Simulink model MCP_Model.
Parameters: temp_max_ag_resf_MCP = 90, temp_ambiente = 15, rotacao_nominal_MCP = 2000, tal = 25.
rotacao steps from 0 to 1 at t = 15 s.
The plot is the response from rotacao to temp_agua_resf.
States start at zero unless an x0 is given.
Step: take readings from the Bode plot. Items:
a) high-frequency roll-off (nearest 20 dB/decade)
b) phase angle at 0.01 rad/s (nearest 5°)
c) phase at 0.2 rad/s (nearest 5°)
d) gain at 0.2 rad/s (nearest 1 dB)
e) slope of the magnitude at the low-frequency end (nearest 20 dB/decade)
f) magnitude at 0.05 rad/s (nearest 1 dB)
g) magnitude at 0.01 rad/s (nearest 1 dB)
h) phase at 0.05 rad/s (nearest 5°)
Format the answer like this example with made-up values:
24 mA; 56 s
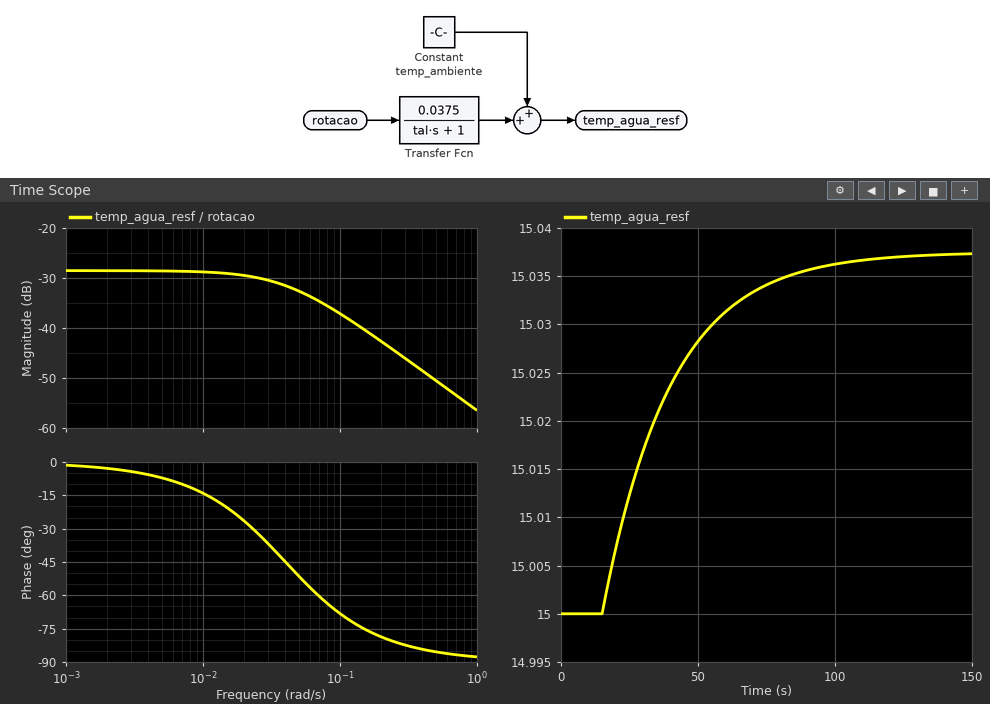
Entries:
-20 dB/decade; -15°; -80°; -43 dB; 0 dB/decade; -33 dB; -29 dB; -50°
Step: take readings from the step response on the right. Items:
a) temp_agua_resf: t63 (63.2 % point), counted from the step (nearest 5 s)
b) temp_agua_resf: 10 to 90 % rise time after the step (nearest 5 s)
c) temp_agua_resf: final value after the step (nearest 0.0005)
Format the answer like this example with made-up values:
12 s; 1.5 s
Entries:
25 s; 55 s; 15.0375
